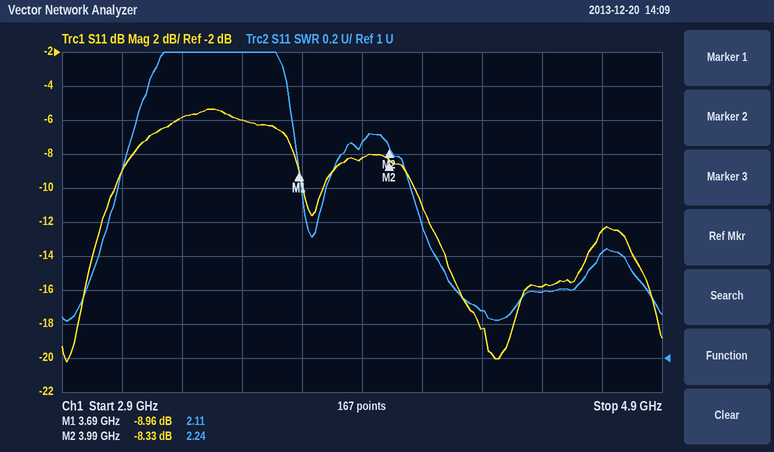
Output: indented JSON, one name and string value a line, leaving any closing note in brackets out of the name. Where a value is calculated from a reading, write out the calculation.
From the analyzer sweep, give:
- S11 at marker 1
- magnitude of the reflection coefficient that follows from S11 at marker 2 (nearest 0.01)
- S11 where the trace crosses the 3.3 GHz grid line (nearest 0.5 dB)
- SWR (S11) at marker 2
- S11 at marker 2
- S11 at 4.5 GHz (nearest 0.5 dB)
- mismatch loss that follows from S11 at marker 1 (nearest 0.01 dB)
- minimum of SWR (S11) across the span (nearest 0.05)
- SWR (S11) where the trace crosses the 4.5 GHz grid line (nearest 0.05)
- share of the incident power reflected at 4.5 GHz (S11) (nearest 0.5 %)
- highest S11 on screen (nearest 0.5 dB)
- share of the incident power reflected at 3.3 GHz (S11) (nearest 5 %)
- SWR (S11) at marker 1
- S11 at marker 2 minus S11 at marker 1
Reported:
{
  "S11 at marker 1": "-8.96 dB",
  "magnitude of the reflection coefficient that follows from S11 at marker 2": "10^(-8.33/20) ≈ 0.38",
  "S11 where the trace crosses the 3.3 GHz grid line": "-6.0 dB",
  "SWR (S11) at marker 2": "2.24",
  "S11 at marker 2": "-8.33 dB",
  "S11 at 4.5 GHz": "-16.0 dB",
  "mismatch loss that follows from S11 at marker 1": "−10 log10(1 − 10^(-8.96/10)) ≈ 0.59 dB",
  "minimum of SWR (S11) across the span": "1.20",
  "SWR (S11) where the trace crosses the 4.5 GHz grid line": "1.40",
  "share of the incident power reflected at 4.5 GHz (S11)": "10^(-16/10) ≈ 2.5 %",
  "highest S11 on screen": "-5.5 dB",
  "share of the incident power reflected at 3.3 GHz (S11)": "10^(-6/10) ≈ 25 %",
  "SWR (S11) at marker 1": "2.11",
  "S11 at marker 2 minus S11 at marker 1": "-8.33 − (-8.96) = 0.63 dB"
}
